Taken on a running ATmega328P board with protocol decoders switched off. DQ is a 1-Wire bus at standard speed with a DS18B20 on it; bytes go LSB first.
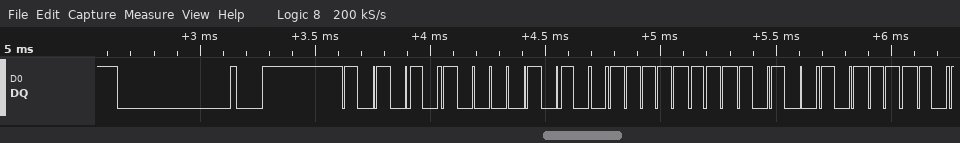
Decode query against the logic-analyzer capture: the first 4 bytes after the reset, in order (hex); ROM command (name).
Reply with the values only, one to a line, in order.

55 28 FF A5
Match ROM
